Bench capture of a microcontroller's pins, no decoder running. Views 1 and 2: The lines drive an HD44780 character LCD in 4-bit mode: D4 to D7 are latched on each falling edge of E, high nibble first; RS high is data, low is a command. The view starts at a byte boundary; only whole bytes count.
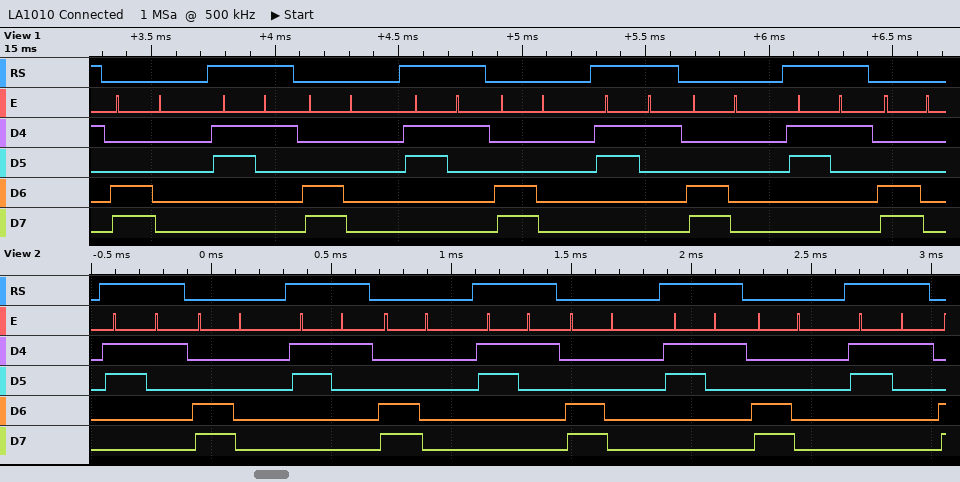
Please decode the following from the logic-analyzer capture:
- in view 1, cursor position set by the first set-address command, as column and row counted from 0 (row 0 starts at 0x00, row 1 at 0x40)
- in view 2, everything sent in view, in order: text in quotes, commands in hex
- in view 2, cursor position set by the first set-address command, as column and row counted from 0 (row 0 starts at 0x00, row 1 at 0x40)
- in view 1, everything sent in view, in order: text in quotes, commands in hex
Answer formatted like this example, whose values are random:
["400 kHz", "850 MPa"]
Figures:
["column 0, row 1", "\"1\" 0xC0 \"1\" 0xC0 \"1\" 0xC0 \"1\" 0xC0 \"1\"", "column 0, row 1", "0xC0 \"1\" 0xC0 \"1\" 0xC0 \"1\" 0xC0 \"1\" 0xC0"]
